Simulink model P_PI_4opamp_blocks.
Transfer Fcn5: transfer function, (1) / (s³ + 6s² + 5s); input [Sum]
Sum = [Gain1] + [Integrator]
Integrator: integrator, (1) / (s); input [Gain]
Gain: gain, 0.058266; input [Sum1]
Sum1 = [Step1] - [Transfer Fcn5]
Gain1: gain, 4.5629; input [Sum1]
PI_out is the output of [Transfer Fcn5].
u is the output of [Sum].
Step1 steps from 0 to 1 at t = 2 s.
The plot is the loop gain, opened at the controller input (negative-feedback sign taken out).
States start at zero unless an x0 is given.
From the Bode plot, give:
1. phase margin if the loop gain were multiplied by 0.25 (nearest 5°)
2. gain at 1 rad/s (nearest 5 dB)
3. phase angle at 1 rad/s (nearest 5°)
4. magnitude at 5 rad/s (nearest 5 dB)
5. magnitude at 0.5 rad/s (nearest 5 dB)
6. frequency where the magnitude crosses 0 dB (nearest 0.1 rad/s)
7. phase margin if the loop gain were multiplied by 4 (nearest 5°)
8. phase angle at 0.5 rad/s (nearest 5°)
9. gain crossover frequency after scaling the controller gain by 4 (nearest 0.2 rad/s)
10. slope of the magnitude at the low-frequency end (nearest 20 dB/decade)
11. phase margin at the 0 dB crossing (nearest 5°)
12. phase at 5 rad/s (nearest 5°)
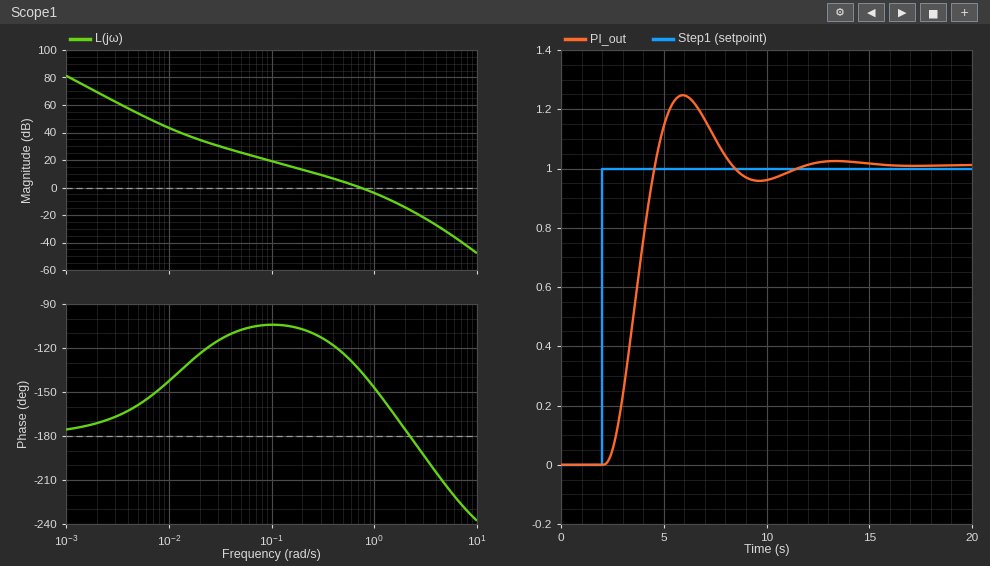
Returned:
70°
-5 dB
-145°
-30 dB
5 dB
0.7 rad/s
10°
-125°
1.8 rad/s
-40 dB/decade
45°
-215°
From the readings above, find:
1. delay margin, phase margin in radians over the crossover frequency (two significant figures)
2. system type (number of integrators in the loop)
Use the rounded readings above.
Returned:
1.1 s
2
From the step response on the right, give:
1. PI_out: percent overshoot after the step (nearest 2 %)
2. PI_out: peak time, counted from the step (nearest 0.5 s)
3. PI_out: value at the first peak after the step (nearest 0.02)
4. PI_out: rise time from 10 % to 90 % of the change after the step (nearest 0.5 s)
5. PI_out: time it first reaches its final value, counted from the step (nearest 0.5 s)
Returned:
24 %
4.0 s
1.24
1.5 s
2.5 s
